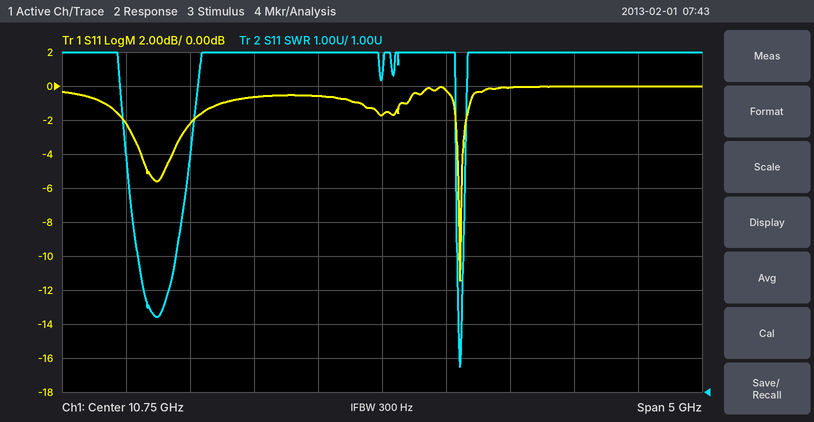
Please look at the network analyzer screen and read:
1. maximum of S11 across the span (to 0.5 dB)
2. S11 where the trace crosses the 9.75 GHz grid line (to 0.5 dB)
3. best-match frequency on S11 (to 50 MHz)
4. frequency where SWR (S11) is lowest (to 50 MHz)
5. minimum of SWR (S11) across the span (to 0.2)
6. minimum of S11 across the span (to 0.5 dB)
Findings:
0.0 dB
-0.5 dB
11.35 GHz
11.35 GHz
1.8
-11.5 dB
